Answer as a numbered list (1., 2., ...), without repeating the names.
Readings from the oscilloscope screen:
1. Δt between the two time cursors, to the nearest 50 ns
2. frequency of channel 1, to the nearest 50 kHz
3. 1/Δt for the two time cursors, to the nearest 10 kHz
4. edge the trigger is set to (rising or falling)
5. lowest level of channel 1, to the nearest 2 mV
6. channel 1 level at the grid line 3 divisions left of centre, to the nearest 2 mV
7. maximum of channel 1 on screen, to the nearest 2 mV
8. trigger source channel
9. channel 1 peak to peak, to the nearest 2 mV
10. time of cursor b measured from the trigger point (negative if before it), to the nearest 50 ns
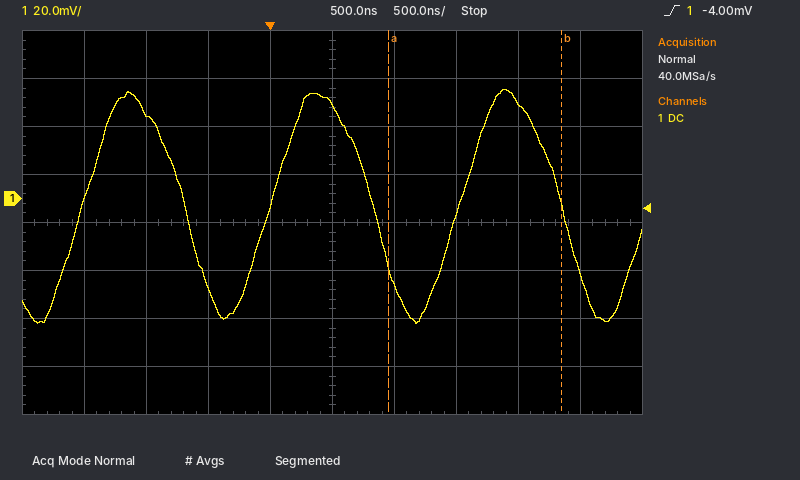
1. 1.40 µs
2. 650 kHz
3. 710 kHz
4. rising
5. -52 mV
6. 36 mV
7. 46 mV
8. channel 1
9. 98 mV
10. +2.35 µs
